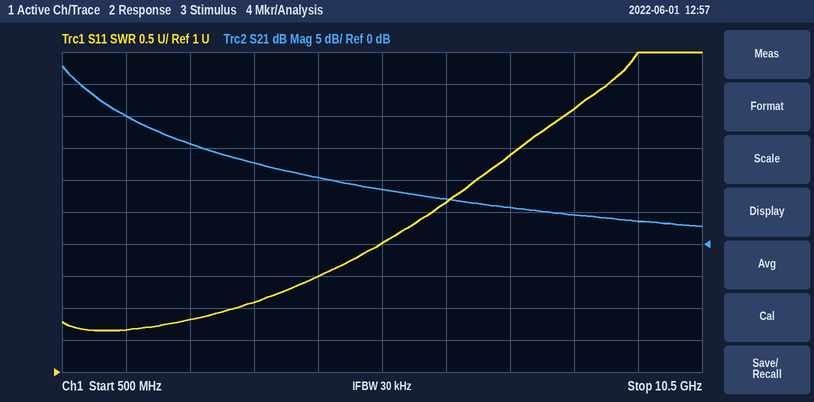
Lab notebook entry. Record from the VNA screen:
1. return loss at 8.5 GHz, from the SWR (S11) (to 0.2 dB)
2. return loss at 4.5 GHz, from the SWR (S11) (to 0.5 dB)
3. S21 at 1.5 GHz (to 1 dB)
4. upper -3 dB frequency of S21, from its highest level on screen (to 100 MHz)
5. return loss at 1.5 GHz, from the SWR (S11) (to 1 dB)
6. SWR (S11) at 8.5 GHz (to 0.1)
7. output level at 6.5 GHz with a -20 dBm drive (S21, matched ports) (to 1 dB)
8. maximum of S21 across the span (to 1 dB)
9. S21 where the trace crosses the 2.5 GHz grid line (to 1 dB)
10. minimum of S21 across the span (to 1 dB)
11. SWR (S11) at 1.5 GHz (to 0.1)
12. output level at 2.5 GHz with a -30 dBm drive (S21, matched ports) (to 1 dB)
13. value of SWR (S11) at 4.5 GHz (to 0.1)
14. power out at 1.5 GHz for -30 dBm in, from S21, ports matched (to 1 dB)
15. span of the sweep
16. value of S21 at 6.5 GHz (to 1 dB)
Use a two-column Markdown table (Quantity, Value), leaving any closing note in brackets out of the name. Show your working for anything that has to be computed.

| Quantity | Value |
|---|---|
| return loss at 8.5 GHz, from the SWR (S11) | −20 log10((5.1 − 1)/(5.1 + 1)) ≈ 3.4 dB |
| return loss at 4.5 GHz, from the SWR (S11) | −20 log10((2.5 − 1)/(2.5 + 1)) ≈ 7.36 dB, so 7.5 dB to the nearest 0.5 dB |
| S21 at 1.5 GHz | 20 dB |
| upper -3 dB frequency of S21, from its highest level on screen | 800 MHz |
| return loss at 1.5 GHz, from the SWR (S11) | −20 log10((1.7 − 1)/(1.7 + 1)) ≈ 12 dB |
| SWR (S11) at 8.5 GHz | 5.1 |
| output level at 6.5 GHz with a -20 dBm drive (S21, matched ports) | -20 dBm + (7 dB) = -13 dBm |
| maximum of S21 across the span | 28 dB |
| S21 where the trace crosses the 2.5 GHz grid line | 16 dB |
| minimum of S21 across the span | 3 dB |
| SWR (S11) at 1.5 GHz | 1.7 |
| output level at 2.5 GHz with a -30 dBm drive (S21, matched ports) | -30 dBm + (16 dB) = -14 dBm |
| value of SWR (S11) at 4.5 GHz | 2.5 |
| power out at 1.5 GHz for -30 dBm in, from S21, ports matched | -30 dBm + (20 dB) = -10 dBm |
| span of the sweep | 10 GHz |
| value of S21 at 6.5 GHz | 7 dB |
